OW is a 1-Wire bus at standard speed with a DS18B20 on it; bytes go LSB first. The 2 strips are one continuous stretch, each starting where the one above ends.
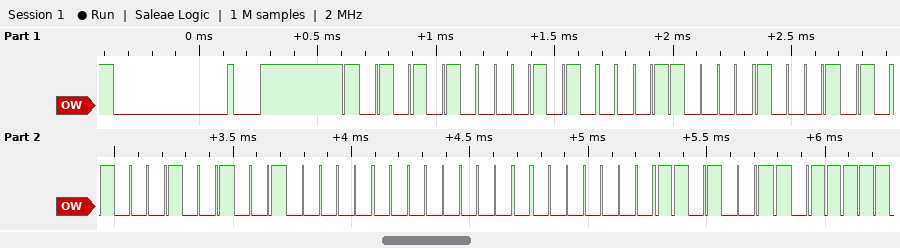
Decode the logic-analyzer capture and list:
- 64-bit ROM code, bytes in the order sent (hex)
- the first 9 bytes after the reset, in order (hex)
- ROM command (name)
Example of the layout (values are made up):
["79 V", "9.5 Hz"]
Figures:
["28 0C 51 91 04 00 00 CB", "55 28 0C 51 91 04 00 00 CB", "Match ROM"]
